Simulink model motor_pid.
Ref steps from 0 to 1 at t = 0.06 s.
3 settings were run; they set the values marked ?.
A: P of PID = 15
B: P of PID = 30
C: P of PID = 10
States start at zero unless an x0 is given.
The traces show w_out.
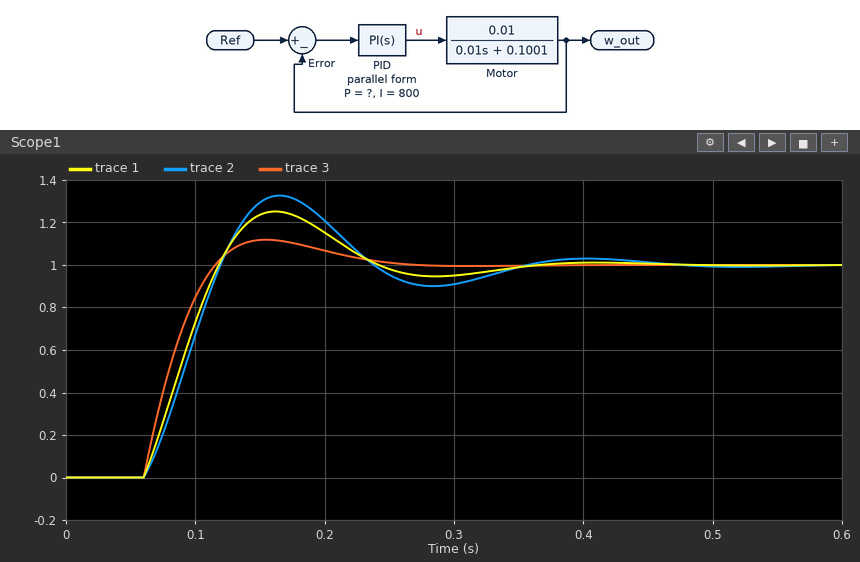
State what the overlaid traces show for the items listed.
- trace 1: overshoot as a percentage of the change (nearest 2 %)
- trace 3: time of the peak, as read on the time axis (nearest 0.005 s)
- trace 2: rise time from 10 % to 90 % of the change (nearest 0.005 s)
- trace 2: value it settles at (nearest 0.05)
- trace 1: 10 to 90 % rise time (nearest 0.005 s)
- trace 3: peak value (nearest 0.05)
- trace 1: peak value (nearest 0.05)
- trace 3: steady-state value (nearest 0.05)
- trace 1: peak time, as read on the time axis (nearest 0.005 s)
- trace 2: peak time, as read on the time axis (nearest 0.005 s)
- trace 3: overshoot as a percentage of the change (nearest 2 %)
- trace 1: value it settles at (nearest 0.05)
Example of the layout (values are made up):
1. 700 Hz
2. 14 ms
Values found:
1. 26 %
2. 0.155 s
3. 0.045 s
4. 1.00
5. 0.045 s
6. 1.10
7. 1.25
8. 1.00
9. 0.160 s
10. 0.165 s
11. 12 %
12. 1.00
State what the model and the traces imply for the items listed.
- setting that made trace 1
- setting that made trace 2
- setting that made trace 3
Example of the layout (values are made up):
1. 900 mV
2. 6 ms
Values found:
1. A
2. C
3. B
